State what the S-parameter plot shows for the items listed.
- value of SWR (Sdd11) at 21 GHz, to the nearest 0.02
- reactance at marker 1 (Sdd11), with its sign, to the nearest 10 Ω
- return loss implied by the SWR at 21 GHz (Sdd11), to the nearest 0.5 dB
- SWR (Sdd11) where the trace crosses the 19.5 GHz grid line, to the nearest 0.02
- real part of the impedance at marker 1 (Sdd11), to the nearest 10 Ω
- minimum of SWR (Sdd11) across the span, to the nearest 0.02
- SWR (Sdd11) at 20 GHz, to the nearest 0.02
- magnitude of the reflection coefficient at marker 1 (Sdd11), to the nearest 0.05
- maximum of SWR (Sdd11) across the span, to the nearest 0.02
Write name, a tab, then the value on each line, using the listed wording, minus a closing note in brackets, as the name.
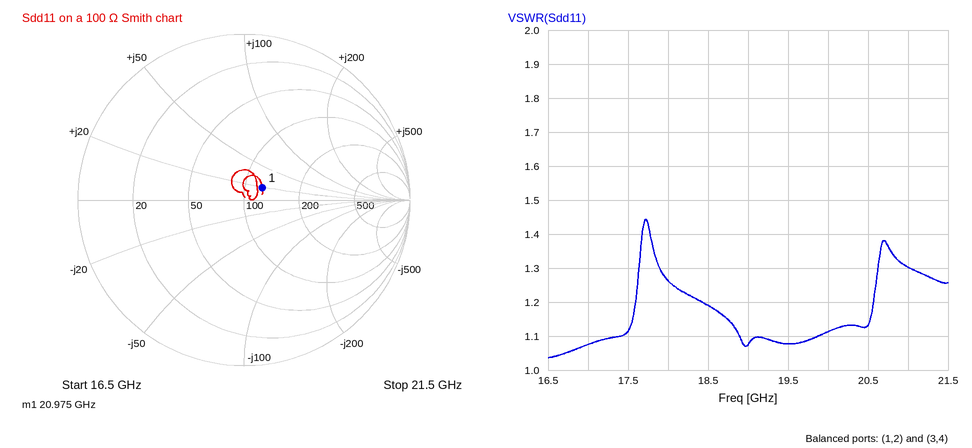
value of SWR (Sdd11) at 21 GHz, to the nearest 0.02	1.30
reactance at marker 1 (Sdd11), with its sign, to the nearest 10 Ω	+20 Ω
return loss implied by the SWR at 21 GHz (Sdd11), to the nearest 0.5 dB	17.5 dB
SWR (Sdd11) where the trace crosses the 19.5 GHz grid line, to the nearest 0.02	1.08
real part of the impedance at marker 1 (Sdd11), to the nearest 10 Ω	120 Ω
minimum of SWR (Sdd11) across the span, to the nearest 0.02	1.04
SWR (Sdd11) at 20 GHz, to the nearest 0.02	1.12
magnitude of the reflection coefficient at marker 1 (Sdd11), to the nearest 0.05	0.15
maximum of SWR (Sdd11) across the span, to the nearest 0.02	1.44
